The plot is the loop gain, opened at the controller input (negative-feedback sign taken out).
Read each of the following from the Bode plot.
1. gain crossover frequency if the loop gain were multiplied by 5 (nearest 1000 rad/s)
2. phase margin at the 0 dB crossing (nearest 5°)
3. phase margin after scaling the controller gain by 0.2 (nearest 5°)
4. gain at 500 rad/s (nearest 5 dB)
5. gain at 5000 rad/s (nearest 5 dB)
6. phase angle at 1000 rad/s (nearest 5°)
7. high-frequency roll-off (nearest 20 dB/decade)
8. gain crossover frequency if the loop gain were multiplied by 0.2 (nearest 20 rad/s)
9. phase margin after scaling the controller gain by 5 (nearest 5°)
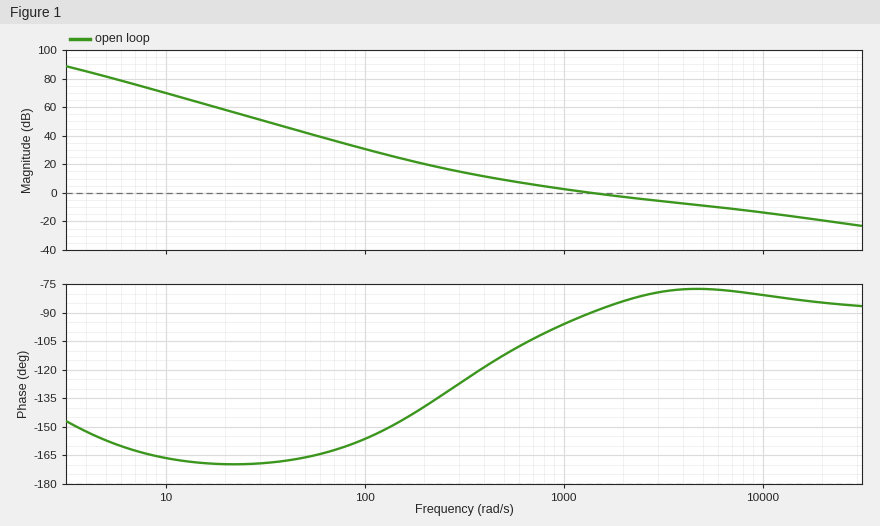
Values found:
10000 rad/s
90°
55°
10 dB
-10 dB
-95°
-20 dB/decade
320 rad/s
100°
